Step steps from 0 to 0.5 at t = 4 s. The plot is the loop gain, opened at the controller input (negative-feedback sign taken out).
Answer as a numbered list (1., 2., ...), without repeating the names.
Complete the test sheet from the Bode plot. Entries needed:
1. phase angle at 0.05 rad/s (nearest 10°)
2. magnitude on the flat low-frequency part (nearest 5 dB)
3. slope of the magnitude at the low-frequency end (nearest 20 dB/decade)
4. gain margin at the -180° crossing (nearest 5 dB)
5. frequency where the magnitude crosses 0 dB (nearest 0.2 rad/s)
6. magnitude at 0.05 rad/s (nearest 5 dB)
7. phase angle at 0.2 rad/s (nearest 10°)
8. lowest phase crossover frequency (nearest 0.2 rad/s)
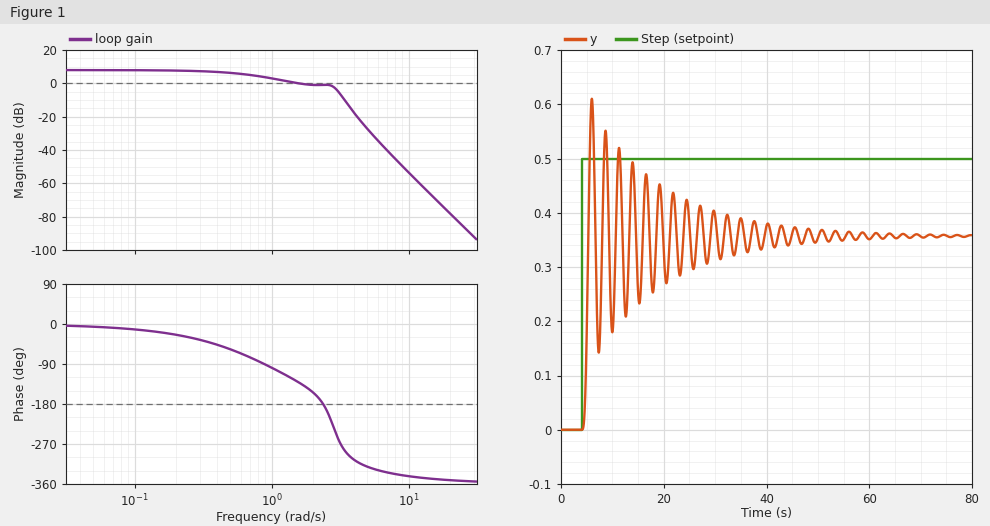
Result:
1. -10°
2. 10 dB
3. 0 dB/decade
4. 0 dB
5. 1.6 rad/s
6. 10 dB
7. -20°
8. 2.4 rad/s
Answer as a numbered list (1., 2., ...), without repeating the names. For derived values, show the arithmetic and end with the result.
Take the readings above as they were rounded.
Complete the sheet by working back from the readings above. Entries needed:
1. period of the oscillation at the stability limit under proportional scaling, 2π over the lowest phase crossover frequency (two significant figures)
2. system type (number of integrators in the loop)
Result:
1. 2π / 2.4 = 2.6 s
2. 0
